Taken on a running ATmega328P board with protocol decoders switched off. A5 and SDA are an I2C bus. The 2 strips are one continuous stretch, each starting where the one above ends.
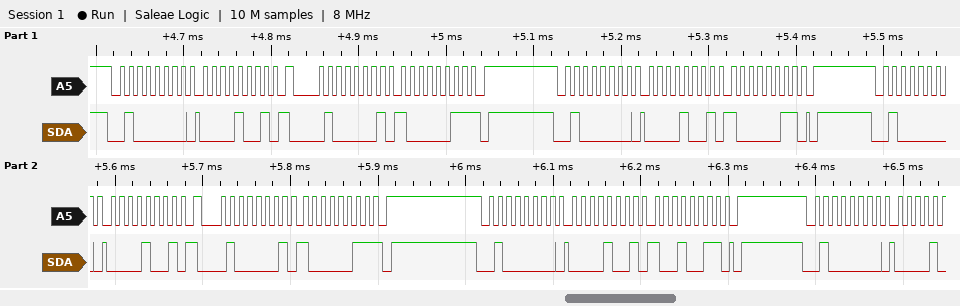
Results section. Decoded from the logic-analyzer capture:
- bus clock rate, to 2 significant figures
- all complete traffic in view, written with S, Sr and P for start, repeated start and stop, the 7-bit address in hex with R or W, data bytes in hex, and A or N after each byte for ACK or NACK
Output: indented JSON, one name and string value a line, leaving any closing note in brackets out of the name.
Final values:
{
  "bus clock rate, to 2 significant figures": "100 kHz",
  "all complete traffic in view, written with S, Sr and P for start, repeated start and stop, the 7-bit address in hex with R or W, data bytes in hex, and A or N after each byte for ACK or NACK": "S 20W A 09 A Sr 20R A 83 N P S 20W A 09 A 83 A P S 20W A 09 A Sr 20R A 83 N P S 20W A 09 A 93 A P S 20W A"
}
